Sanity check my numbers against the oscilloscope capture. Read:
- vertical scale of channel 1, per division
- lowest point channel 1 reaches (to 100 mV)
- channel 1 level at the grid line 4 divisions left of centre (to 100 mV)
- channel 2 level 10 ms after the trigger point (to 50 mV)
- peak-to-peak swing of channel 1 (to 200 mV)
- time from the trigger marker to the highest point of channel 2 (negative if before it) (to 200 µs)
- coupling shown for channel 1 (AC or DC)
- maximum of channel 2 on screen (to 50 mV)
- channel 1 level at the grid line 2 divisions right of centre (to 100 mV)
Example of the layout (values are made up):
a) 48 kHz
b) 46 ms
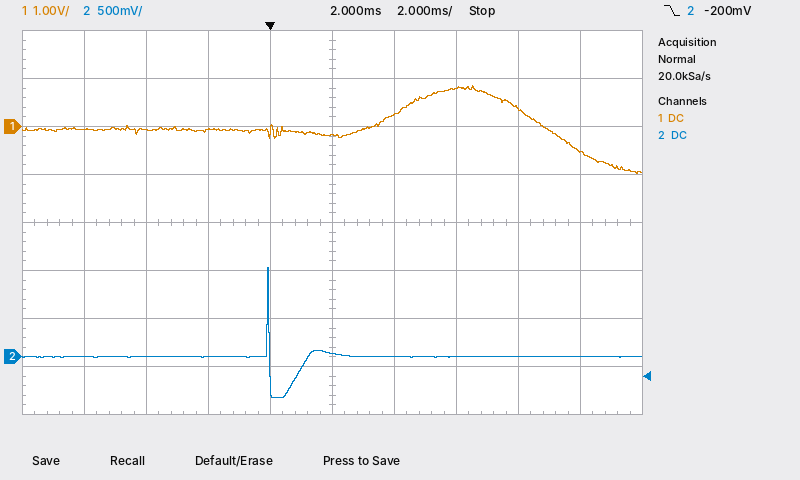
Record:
a) 1 V
b) -1.0 V
c) -100 mV
d) 0 mV
e) 1.8 V
f) 0.0 ms
g) DC
h) 950 mV
i) 800 mV
